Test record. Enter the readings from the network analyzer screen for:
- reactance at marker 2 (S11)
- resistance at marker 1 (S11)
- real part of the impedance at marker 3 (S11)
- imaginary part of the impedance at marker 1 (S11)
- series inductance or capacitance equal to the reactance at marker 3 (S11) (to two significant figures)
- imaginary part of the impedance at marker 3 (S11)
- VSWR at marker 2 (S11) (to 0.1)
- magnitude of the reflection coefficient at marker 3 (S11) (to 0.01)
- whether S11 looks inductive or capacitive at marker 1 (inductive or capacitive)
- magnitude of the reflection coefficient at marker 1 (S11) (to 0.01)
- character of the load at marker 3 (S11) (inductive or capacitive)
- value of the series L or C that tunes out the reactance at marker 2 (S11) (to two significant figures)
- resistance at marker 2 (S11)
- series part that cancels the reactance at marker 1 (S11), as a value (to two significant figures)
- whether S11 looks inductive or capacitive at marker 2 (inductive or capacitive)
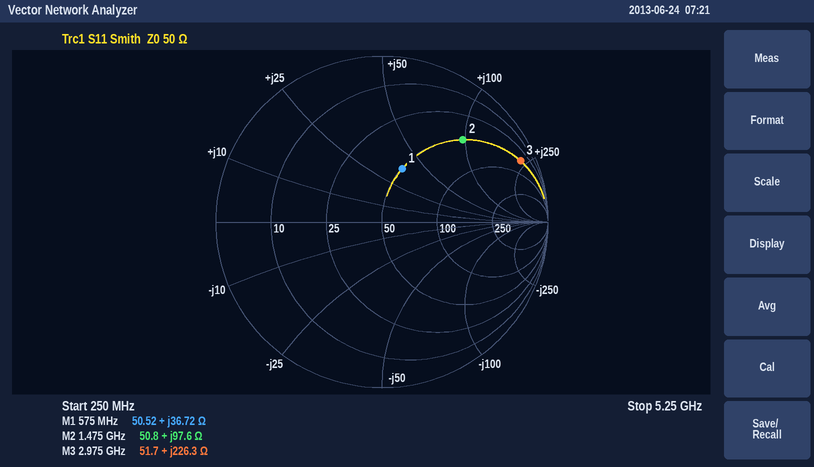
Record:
+97.6 Ω
50.52 Ω
51.7 Ω
+36.72 Ω
12 nH
+226.3 Ω
5.6
0.91
inductive
0.34
inductive
1.1 pF
50.8 Ω
7.5 pF
inductive
